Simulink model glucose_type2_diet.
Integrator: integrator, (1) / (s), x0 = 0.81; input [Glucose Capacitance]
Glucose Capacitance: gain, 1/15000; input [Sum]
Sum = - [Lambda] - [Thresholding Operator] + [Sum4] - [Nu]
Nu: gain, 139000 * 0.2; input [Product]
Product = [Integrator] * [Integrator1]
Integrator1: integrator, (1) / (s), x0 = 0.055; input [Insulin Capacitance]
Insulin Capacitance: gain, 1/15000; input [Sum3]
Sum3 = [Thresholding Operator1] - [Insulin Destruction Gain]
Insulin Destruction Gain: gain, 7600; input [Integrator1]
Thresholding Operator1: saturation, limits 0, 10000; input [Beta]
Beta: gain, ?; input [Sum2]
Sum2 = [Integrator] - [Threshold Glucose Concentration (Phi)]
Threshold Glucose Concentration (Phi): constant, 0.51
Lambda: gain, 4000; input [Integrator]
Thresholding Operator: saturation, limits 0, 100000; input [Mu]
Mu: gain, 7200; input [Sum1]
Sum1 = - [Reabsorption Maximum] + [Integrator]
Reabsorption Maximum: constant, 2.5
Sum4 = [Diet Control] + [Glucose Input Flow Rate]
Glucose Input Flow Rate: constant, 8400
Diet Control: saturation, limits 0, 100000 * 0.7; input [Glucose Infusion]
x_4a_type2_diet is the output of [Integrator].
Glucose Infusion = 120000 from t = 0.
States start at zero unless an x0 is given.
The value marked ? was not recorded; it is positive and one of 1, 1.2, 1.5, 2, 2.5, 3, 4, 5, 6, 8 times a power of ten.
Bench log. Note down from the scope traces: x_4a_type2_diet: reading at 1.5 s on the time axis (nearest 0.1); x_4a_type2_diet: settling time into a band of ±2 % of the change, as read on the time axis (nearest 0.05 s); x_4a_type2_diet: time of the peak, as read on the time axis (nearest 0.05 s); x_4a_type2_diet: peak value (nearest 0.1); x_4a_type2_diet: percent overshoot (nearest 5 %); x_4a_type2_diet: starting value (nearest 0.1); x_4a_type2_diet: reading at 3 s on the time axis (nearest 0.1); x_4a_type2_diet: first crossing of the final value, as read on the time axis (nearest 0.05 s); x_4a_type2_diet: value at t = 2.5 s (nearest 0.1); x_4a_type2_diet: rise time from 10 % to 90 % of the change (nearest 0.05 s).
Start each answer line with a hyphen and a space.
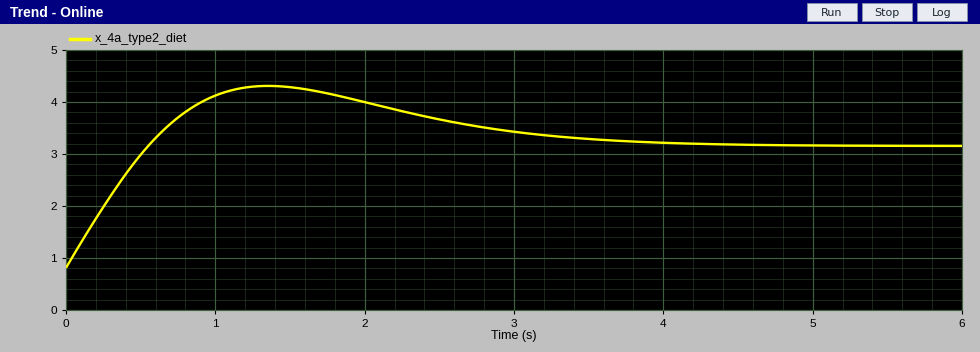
- 4.3
- 4.15 s
- 1.35 s
- 4.3
- 50 %
- 0.8
- 3.4
- 0.55 s
- 3.7
- 0.45 s
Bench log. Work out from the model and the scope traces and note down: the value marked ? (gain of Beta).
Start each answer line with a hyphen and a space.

- 2000
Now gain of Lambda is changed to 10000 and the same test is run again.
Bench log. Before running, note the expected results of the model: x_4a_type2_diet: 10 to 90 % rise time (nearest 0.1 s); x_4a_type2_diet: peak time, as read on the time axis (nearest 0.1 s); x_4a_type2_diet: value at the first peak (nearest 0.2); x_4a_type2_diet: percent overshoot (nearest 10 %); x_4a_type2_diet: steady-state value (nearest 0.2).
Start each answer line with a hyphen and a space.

- 0.4 s
- 1.3 s
- 3.6
- 40 %
- 2.8
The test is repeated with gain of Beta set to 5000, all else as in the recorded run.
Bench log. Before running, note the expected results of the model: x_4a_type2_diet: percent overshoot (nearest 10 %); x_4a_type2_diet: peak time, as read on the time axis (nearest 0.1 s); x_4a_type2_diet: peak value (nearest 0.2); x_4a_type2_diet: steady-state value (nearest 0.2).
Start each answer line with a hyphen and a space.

- 100 %
- 1.1 s
- 3.6
- 2.2
